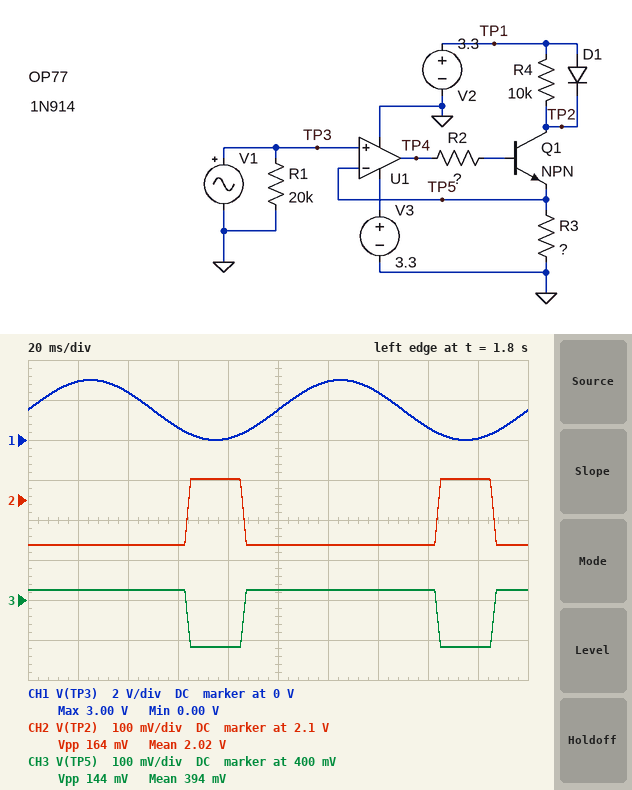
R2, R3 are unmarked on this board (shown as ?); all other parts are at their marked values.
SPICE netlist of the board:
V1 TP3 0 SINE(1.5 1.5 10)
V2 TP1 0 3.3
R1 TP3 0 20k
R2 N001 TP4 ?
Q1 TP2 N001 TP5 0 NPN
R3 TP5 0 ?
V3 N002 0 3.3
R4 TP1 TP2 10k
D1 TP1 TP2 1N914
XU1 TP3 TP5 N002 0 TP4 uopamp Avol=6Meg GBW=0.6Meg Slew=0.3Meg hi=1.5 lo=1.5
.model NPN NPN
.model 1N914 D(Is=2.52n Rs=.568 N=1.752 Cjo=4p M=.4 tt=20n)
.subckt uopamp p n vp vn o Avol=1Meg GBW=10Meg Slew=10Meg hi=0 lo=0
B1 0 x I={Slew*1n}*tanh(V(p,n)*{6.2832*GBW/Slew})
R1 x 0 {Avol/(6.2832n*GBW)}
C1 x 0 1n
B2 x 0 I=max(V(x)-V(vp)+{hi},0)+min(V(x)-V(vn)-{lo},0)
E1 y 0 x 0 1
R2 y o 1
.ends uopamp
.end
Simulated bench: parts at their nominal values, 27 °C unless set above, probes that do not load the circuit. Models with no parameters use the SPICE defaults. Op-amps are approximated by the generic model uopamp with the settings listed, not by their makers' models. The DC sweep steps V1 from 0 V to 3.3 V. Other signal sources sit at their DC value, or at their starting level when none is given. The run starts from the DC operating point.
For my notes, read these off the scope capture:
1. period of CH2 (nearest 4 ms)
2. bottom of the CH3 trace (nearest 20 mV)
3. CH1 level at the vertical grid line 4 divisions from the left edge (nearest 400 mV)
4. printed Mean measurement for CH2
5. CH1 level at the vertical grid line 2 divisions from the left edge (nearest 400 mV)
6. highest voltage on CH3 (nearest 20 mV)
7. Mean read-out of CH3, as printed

100 ms
280 mV
0 V
2.02 V
2.4 V
420 mV
394 mV
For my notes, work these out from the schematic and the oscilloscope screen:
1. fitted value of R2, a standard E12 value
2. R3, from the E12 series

56 Ω
0.56 Ω
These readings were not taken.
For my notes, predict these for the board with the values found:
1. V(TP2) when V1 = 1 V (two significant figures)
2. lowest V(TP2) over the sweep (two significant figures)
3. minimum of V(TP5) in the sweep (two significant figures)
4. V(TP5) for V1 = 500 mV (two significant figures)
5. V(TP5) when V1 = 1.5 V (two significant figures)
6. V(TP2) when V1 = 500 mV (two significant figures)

2.0 V
2.0 V
280 mV
430 mV
430 mV
2.0 V
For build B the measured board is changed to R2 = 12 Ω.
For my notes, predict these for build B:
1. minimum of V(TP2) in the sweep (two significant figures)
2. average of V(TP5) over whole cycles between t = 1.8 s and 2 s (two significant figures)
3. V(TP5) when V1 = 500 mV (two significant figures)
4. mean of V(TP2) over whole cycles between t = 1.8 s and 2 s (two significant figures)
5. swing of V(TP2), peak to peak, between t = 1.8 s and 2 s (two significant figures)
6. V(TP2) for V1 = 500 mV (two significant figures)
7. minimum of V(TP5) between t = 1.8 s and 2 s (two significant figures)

1.7 V
620 mV
500 mV
1.8 V
260 mV
1.9 V
450 mV
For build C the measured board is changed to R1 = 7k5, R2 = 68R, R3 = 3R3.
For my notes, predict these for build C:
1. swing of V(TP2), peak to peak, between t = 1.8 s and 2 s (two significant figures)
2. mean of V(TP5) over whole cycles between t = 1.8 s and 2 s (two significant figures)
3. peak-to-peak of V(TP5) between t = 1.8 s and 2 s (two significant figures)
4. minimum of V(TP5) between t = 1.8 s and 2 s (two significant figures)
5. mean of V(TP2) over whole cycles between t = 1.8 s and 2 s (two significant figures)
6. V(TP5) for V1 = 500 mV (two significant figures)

59 mV
660 mV
240 mV
490 mV
2.4 V
500 mV
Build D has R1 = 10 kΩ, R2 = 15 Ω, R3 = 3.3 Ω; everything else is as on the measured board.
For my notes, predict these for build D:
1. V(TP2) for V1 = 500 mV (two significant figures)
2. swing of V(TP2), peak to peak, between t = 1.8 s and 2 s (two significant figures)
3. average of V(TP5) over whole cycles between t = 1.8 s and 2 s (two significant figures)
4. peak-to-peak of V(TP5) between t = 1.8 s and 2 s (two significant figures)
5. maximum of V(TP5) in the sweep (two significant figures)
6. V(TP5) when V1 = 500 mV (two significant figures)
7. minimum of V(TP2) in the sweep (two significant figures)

2.4 V
65 mV
750 mV
280 mV
840 mV
570 mV
2.3 V
